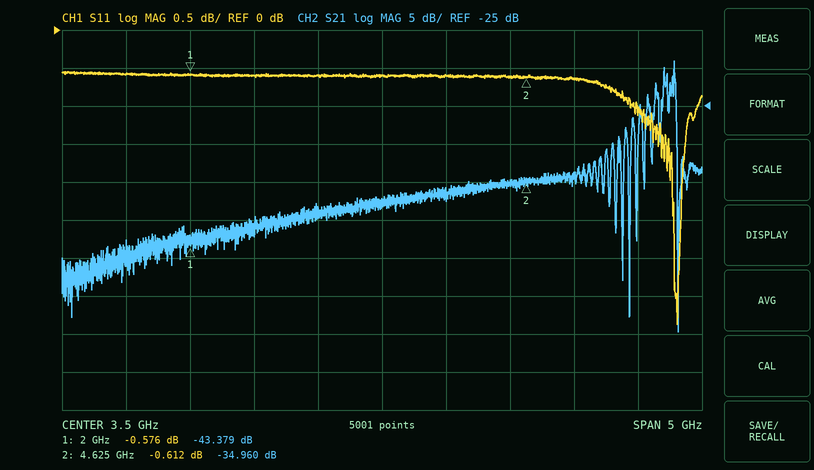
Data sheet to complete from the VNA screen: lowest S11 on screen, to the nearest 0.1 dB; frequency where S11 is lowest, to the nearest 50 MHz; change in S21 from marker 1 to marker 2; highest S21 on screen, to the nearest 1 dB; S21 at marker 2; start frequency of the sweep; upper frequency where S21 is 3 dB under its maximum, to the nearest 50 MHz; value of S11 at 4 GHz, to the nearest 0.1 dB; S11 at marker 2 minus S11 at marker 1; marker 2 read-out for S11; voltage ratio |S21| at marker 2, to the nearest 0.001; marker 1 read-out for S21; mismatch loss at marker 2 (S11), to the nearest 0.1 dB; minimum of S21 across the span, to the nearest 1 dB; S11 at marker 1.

-3.9 dB
5.80 GHz
8.419 dB
-19 dB
-34.960 dB
1 GHz
5.80 GHz
-0.6 dB
-0.036 dB
-0.612 dB
0.018
-43.379 dB
8.8 dB
-55 dB
-0.576 dB
